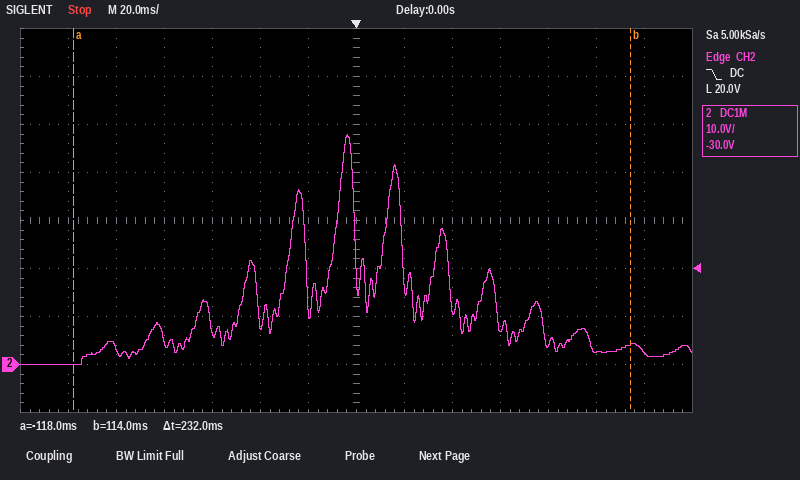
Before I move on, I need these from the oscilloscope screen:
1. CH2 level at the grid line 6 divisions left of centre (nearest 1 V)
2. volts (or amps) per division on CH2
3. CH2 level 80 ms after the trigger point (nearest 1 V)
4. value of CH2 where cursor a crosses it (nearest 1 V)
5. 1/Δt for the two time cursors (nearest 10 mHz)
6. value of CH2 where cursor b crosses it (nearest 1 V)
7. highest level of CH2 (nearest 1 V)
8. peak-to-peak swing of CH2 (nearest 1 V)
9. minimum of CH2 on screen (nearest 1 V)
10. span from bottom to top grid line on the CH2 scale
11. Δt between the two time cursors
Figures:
0 V
10 V
4 V
0 V
4.31 Hz
4 V
48 V
48 V
0 V
80 V
232 ms
